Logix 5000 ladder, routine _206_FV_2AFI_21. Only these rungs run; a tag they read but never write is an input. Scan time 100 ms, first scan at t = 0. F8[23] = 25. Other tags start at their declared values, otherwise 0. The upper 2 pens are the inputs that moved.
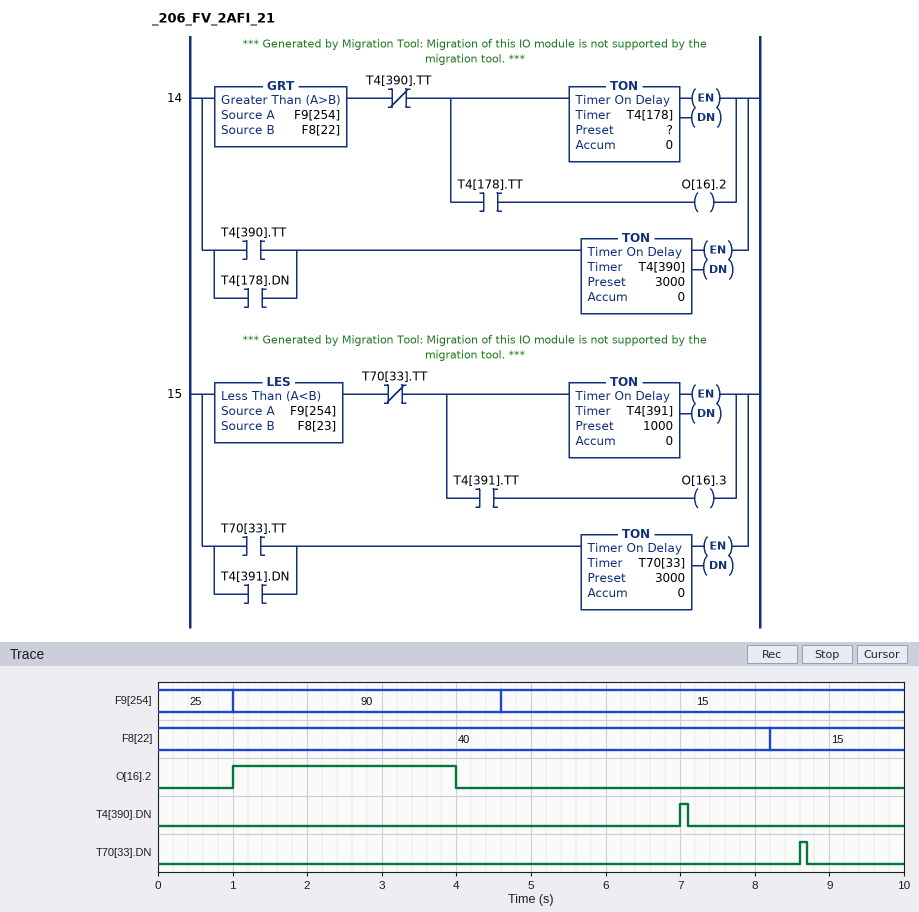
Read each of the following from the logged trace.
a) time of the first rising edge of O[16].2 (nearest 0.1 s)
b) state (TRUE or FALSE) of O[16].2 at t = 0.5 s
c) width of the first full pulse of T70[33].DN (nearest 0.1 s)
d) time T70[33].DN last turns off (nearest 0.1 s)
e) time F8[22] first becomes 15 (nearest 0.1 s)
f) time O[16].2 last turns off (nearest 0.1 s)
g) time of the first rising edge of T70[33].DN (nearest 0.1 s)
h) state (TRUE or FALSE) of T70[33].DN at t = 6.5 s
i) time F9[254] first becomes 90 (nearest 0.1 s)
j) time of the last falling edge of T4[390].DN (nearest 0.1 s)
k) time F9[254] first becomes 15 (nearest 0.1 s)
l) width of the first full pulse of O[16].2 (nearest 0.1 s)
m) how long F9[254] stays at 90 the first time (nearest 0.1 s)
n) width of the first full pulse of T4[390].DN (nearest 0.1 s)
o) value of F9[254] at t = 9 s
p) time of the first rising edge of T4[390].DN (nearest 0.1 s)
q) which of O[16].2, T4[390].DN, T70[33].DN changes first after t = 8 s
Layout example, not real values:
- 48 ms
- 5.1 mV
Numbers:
- 1.0 s
- FALSE
- 0.1 s
- 8.7 s
- 8.2 s
- 4.0 s
- 8.6 s
- FALSE
- 1.0 s
- 7.1 s
- 4.6 s
- 3.0 s
- 3.6 s
- 0.1 s
- 15
- 7.0 s
- T70[33].DN
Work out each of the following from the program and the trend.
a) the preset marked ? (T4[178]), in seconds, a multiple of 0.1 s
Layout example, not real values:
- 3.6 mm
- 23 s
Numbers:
- 3.0 s
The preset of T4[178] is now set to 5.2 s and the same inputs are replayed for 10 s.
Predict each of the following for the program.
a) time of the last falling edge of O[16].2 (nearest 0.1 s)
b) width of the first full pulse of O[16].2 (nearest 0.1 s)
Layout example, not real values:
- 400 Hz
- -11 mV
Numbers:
- 4.6 s
- 3.6 s
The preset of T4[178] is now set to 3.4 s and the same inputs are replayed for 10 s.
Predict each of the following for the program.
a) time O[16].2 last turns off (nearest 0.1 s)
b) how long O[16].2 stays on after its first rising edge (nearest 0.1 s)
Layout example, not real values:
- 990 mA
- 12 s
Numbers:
- 4.4 s
- 3.4 s
